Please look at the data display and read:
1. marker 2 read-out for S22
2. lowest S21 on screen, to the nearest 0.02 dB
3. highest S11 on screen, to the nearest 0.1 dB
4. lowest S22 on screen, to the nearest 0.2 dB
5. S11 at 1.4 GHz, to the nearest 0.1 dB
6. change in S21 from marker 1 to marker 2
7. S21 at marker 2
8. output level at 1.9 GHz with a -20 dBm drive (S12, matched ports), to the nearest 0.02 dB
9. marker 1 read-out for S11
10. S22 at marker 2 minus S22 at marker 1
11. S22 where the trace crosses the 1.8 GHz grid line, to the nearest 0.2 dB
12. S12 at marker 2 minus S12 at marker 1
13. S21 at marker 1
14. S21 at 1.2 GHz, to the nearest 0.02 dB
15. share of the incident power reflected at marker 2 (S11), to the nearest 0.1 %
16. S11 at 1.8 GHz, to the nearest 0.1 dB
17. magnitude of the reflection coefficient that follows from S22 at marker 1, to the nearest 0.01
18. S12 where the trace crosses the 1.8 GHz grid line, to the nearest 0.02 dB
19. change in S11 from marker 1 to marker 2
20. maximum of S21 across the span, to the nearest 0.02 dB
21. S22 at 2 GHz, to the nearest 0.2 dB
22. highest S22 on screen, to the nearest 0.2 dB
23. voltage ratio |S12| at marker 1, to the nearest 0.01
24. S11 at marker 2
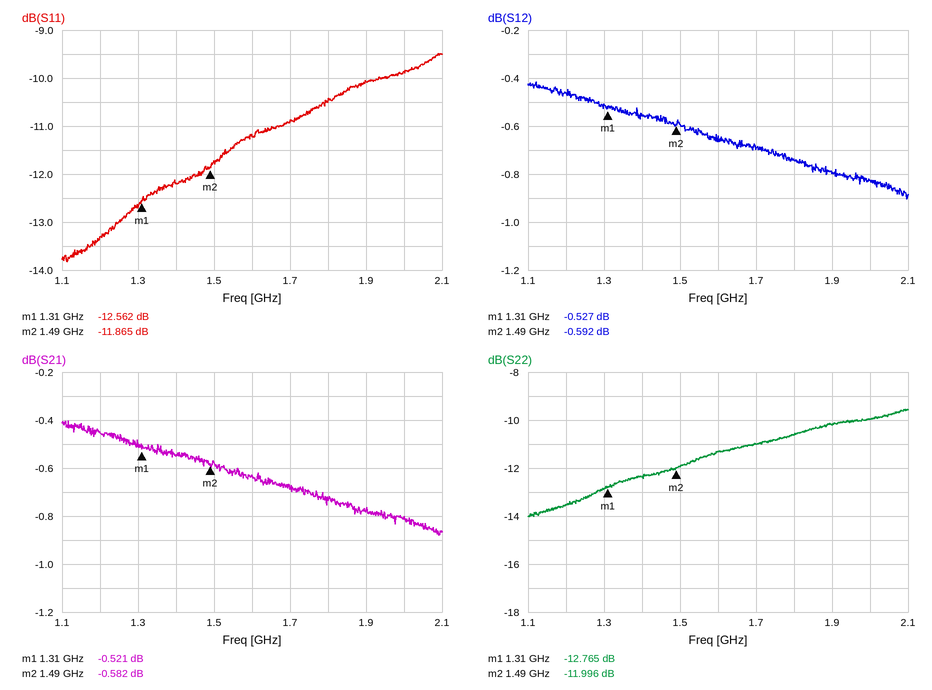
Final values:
-11.996 dB
-0.88 dB
-9.5 dB
-14.0 dB
-12.2 dB
-0.061 dB
-0.582 dB
-20.80 dBm
-12.562 dB
0.769 dB
-10.6 dB
-0.065 dB
-0.521 dB
-0.46 dB
6.5 %
-10.5 dB
0.23
-0.74 dB
0.697 dB
-0.40 dB
-10.0 dB
-9.6 dB
0.94
-11.865 dB
